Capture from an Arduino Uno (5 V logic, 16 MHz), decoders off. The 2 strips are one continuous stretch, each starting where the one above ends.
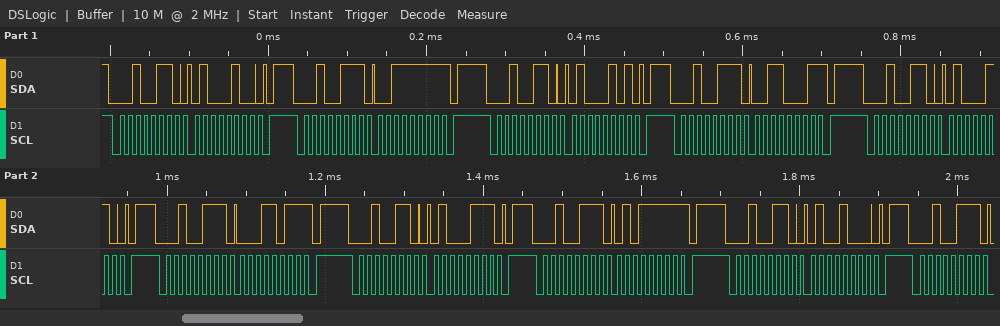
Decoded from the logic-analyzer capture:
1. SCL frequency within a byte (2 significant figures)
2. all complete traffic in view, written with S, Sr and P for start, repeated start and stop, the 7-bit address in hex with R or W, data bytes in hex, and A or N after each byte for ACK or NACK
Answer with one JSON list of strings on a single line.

["100 kHz", "S 13W A 44 A P S 13R A 3F N P S 13W A 45 A P S 13R A 31 N P S 13W A 46 A P S 13R A 1B N P S 13W A 47 A P S 13R A 5F N P S 13W A 48 A P S 13R A"]
